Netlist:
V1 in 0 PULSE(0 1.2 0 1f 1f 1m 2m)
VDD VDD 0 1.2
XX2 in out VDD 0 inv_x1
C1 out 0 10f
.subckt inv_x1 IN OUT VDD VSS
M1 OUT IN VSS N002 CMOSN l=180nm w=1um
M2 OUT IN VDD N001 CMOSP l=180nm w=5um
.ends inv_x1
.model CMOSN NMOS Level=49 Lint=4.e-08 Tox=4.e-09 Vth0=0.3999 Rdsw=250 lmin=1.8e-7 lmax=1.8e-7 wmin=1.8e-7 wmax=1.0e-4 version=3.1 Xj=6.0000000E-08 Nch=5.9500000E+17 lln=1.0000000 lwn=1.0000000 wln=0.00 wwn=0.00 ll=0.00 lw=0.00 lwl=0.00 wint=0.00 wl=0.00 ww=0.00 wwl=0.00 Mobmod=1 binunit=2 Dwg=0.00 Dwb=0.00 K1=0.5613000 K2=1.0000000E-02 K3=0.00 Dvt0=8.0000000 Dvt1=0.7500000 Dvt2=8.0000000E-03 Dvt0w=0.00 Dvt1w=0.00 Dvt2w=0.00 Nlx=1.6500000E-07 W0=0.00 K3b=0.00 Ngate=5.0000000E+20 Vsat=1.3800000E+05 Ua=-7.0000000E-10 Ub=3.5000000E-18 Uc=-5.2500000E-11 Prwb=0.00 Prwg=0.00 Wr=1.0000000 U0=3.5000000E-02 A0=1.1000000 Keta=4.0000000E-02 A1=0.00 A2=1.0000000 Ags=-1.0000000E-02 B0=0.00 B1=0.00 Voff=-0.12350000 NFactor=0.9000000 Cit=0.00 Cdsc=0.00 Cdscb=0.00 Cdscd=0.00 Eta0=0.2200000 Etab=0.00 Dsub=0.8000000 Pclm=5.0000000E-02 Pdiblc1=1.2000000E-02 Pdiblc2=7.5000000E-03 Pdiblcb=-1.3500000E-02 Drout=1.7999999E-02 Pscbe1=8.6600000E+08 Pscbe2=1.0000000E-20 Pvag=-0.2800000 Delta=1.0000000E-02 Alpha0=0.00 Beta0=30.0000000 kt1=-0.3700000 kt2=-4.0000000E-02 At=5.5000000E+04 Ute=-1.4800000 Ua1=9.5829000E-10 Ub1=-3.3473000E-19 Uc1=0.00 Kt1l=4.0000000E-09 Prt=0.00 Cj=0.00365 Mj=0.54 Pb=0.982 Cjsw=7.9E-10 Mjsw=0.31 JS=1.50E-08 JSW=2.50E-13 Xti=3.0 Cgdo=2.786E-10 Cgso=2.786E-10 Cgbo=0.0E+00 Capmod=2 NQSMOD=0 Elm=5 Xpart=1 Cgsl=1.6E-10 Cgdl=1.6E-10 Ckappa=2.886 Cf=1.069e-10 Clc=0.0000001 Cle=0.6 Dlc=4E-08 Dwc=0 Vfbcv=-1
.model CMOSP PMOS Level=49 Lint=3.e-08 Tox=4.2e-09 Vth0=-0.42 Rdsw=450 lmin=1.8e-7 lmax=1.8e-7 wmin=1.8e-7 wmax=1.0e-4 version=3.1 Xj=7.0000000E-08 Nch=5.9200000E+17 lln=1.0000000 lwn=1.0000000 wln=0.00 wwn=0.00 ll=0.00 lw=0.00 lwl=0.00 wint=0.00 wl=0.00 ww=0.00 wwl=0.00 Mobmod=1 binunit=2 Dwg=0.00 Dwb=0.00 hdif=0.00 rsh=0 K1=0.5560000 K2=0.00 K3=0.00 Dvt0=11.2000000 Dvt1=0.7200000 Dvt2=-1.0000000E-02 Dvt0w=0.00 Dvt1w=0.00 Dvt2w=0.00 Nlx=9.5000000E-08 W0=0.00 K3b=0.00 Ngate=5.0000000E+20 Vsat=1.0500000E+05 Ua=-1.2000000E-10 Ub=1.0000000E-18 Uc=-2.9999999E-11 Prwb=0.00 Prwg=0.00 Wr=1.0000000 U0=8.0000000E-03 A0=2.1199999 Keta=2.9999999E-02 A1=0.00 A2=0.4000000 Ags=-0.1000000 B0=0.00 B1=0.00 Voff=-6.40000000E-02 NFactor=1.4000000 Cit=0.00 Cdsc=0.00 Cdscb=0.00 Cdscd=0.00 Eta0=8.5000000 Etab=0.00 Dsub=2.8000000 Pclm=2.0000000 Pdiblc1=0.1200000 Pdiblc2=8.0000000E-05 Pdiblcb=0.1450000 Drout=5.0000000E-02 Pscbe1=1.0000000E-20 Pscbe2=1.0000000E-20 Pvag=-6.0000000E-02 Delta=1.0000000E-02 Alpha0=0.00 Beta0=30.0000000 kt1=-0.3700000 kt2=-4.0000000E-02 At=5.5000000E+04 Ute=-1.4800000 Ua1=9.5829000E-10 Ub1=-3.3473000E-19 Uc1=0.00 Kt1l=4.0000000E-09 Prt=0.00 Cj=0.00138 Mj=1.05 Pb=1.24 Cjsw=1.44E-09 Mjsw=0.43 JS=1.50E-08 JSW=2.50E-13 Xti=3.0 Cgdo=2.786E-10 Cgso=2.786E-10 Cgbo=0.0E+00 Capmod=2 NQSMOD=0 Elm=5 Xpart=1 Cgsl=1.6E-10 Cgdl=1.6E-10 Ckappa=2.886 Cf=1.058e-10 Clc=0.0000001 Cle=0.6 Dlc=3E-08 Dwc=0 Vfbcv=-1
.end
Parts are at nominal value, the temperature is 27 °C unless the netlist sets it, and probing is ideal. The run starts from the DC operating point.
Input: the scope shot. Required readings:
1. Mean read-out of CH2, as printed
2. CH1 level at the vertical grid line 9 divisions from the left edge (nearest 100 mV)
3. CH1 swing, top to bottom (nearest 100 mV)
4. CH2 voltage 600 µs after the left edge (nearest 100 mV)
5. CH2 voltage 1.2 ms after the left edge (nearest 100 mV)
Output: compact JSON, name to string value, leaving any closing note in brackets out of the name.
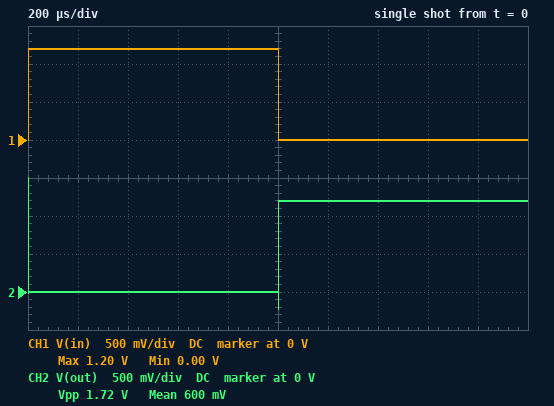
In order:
{"Mean read-out of CH2, as printed": "600 mV", "CH1 level at the vertical grid line 9 divisions from the left edge": "0 V", "CH1 swing, top to bottom": "1.2 V", "CH2 voltage 600 µs after the left edge": "0 V", "CH2 voltage 1.2 ms after the left edge": "1.2 V"}
